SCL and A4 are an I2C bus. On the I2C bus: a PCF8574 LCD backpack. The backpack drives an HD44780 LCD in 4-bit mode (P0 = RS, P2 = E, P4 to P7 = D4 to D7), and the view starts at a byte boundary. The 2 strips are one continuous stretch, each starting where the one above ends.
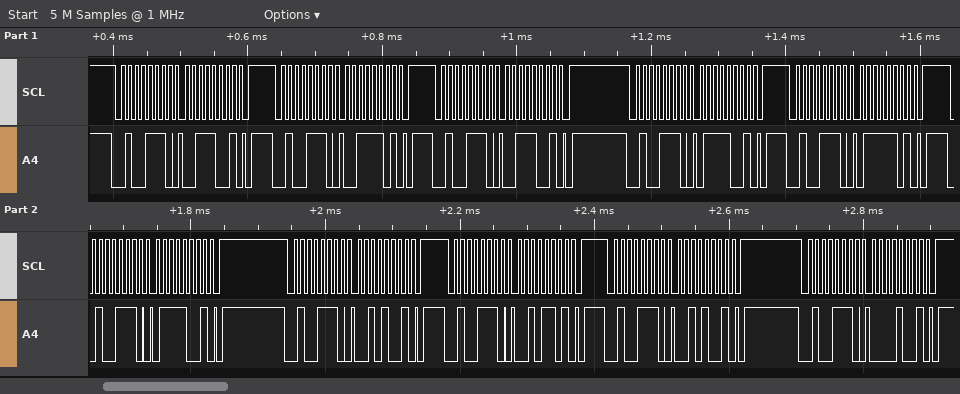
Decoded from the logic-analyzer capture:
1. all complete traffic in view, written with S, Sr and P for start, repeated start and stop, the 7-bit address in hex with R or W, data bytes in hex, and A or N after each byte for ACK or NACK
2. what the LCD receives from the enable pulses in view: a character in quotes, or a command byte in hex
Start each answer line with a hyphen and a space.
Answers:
- S 27W A 39 A P S 27W A 3D A P S 27W A 39 A P S 27W A 79 A P S 27W A 7D A P S 27W A 79 A P S 27W A 29 A P S 27W A 2D A P S 27W A 29 A P S 27W A 09 A P
- '7'
